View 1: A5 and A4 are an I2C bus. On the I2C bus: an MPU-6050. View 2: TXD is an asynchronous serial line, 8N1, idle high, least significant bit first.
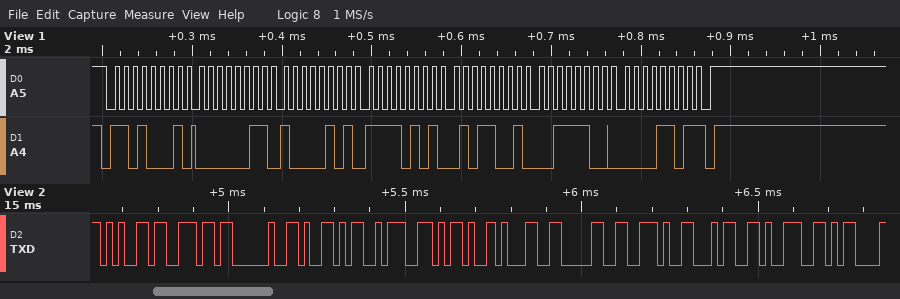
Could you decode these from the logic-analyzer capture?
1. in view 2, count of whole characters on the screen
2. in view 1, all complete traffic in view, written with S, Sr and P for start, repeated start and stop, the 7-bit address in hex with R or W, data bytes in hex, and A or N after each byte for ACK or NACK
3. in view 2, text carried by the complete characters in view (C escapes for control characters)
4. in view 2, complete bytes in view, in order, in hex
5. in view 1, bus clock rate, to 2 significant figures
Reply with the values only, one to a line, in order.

12
S 68R A 03 A 85 A F5 A 59 A 3C A 0D N P
"en Y:-10.49\r"
65 6E 20 59 3A 2D 31 30 2E 34 39 0D
100 kHz
